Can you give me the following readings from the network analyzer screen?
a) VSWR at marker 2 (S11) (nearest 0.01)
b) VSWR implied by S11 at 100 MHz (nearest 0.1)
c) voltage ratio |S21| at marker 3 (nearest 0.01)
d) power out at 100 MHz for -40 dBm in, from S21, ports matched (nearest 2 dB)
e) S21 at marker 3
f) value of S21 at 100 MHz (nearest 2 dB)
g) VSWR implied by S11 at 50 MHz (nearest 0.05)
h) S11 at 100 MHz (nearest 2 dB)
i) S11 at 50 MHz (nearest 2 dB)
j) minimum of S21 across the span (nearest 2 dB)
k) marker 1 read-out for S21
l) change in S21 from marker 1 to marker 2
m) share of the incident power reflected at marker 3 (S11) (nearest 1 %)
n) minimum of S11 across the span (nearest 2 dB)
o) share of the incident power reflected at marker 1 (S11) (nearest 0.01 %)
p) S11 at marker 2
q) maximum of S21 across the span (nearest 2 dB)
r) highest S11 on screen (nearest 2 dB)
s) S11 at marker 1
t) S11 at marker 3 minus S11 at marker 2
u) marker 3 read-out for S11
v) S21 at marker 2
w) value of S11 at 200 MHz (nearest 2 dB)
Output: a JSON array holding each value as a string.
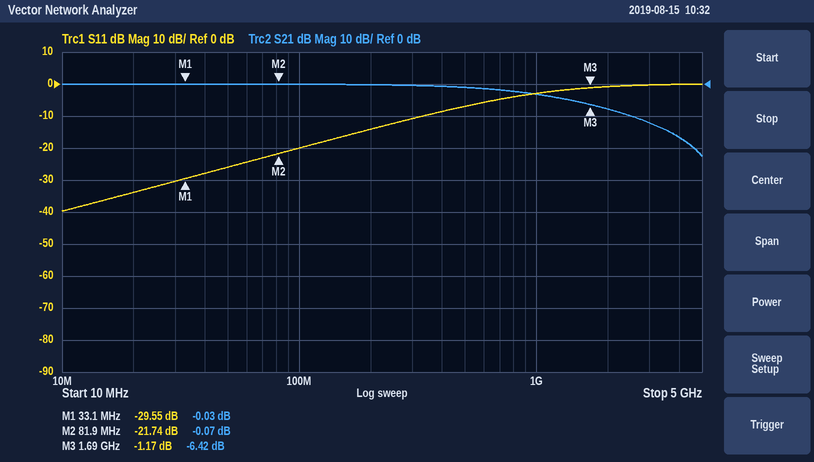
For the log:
["1.18", "1.2", "0.48", "-40 dBm", "-6.42 dB", "0 dB", "1.10", "-20 dB", "-26 dB", "-22 dB", "-0.03 dB", "-0.04 dB", "76 %", "-40 dB", "0.11 %", "-21.74 dB", "0 dB", "0 dB", "-29.55 dB", "20.57 dB", "-1.17 dB", "-0.07 dB", "-14 dB"]
